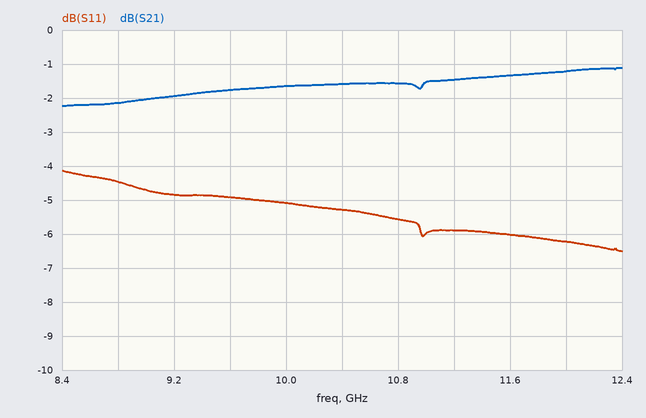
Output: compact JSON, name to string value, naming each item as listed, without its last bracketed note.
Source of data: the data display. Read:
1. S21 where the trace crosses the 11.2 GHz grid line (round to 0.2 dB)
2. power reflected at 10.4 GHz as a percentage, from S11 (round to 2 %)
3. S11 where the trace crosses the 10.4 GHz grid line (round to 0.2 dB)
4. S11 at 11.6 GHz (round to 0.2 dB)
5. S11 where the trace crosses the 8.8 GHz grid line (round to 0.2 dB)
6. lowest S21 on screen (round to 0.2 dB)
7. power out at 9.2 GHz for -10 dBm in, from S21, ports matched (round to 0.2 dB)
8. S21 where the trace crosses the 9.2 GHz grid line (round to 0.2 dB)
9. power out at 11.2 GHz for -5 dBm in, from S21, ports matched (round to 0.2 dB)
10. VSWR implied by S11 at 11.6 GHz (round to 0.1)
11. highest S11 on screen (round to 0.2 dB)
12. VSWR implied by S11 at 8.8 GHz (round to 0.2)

{"S21 where the trace crosses the 11.2 GHz grid line": "-1.4 dB", "power reflected at 10.4 GHz as a percentage, from S11": "30 %", "S11 where the trace crosses the 10.4 GHz grid line": "-5.2 dB", "S11 at 11.6 GHz": "-6.0 dB", "S11 where the trace crosses the 8.8 GHz grid line": "-4.4 dB", "lowest S21 on screen": "-2.2 dB", "power out at 9.2 GHz for -10 dBm in, from S21, ports matched": "-12.0 dBm", "S21 where the trace crosses the 9.2 GHz grid line": "-2.0 dB", "power out at 11.2 GHz for -5 dBm in, from S21, ports matched": "-6.4 dBm", "VSWR implied by S11 at 11.6 GHz": "3.0", "highest S11 on screen": "-4.2 dB", "VSWR implied by S11 at 8.8 GHz": "4.0"}
